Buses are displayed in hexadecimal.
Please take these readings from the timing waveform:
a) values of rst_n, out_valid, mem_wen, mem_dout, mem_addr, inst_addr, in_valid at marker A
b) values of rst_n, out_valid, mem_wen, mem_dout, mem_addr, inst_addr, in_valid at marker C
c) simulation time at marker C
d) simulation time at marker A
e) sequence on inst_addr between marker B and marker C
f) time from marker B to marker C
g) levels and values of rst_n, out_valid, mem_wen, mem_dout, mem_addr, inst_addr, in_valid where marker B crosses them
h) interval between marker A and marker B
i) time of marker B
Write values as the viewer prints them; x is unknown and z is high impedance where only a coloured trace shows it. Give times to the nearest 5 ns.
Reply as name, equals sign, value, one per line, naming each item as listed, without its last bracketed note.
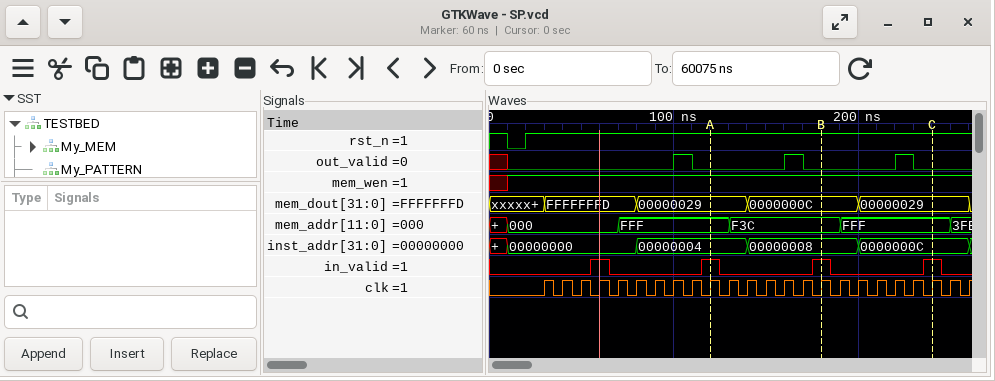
values of rst_n, out_valid, mem_wen, mem_dout, mem_addr, inst_addr, in_valid at marker A = rst_n=1, out_valid=0, mem_wen=1, mem_dout=00000029, mem_addr=FFF, inst_addr=00000004, in_valid=1
values of rst_n, out_valid, mem_wen, mem_dout, mem_addr, inst_addr, in_valid at marker C = rst_n=1, out_valid=0, mem_wen=1, mem_dout=00000029, mem_addr=FFF, inst_addr=0000000C, in_valid=1
simulation time at marker C = 240 ns
simulation time at marker A = 120 ns
sequence on inst_addr between marker B and marker C = 00000008, 0000000C
time from marker B to marker C = 60 ns
levels and values of rst_n, out_valid, mem_wen, mem_dout, mem_addr, inst_addr, in_valid where marker B crosses them = rst_n=1, out_valid=0, mem_wen=1, mem_dout=0000000C, mem_addr=F3C, inst_addr=00000008, in_valid=1
interval between marker A and marker B = 60 ns
time of marker B = 180 ns
